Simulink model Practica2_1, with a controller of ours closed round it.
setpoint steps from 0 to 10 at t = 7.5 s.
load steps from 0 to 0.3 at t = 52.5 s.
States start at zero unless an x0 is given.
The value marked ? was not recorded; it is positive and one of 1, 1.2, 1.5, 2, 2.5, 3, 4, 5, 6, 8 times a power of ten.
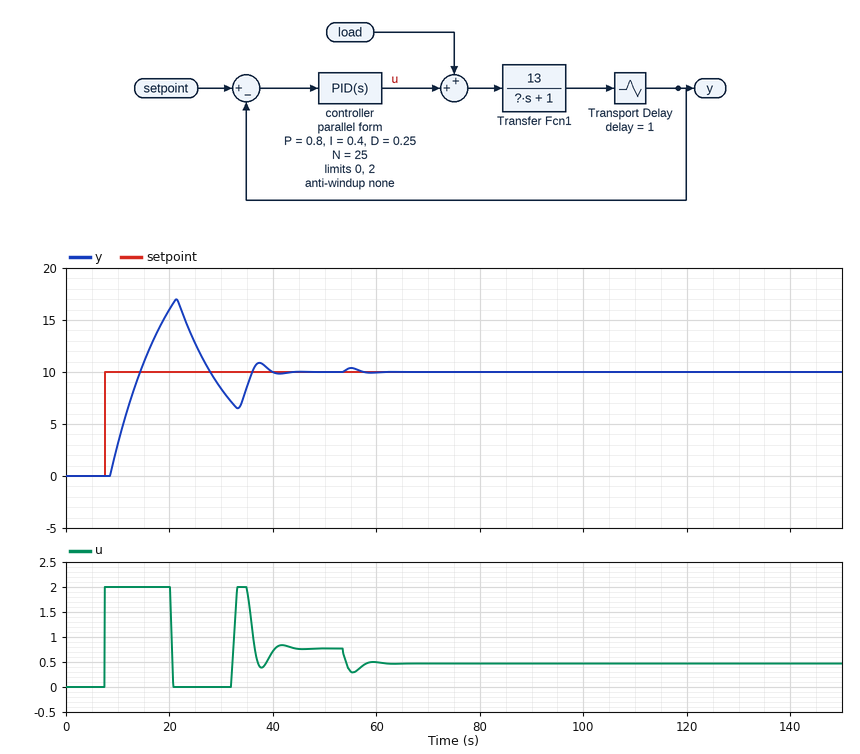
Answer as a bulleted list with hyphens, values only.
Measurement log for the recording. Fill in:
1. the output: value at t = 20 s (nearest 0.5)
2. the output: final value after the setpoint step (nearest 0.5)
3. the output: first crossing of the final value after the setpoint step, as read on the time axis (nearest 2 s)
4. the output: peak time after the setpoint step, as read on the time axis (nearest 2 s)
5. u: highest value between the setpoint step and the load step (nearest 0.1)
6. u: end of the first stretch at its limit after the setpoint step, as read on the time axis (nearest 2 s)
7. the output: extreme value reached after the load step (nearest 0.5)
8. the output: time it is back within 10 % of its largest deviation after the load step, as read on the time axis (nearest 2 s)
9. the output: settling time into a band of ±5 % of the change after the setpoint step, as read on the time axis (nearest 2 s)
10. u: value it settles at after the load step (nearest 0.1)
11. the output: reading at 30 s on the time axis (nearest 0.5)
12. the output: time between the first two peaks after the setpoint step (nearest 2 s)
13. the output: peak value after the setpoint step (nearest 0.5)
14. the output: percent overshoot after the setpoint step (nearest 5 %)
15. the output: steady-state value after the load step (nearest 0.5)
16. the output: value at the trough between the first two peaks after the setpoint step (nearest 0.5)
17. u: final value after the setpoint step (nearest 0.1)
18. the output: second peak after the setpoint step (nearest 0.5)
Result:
- 16.0
- 10.0
- 14 s
- 22 s
- 2.0
- 20 s
- 10.5
- 60 s
- 38 s
- 0.5
- 8.5
- 16 s
- 17.0
- 70 %
- 10.0
- 6.5
- 0.8
- 11.0
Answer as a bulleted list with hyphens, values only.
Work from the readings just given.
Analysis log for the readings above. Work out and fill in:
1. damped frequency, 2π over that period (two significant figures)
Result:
- 0.39 rad/s
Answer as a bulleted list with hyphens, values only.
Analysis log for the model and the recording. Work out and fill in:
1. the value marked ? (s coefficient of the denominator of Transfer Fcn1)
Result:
- 12
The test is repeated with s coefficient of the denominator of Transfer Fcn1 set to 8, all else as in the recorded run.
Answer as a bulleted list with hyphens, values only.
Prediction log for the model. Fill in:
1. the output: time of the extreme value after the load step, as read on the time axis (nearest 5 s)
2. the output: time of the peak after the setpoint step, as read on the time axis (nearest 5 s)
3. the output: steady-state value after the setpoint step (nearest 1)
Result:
- 55 s
- 15 s
- 10
